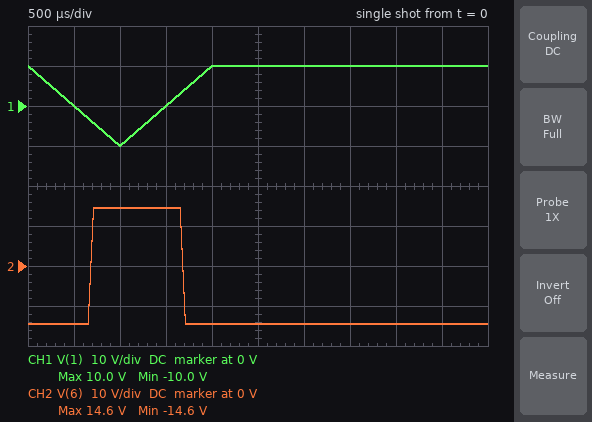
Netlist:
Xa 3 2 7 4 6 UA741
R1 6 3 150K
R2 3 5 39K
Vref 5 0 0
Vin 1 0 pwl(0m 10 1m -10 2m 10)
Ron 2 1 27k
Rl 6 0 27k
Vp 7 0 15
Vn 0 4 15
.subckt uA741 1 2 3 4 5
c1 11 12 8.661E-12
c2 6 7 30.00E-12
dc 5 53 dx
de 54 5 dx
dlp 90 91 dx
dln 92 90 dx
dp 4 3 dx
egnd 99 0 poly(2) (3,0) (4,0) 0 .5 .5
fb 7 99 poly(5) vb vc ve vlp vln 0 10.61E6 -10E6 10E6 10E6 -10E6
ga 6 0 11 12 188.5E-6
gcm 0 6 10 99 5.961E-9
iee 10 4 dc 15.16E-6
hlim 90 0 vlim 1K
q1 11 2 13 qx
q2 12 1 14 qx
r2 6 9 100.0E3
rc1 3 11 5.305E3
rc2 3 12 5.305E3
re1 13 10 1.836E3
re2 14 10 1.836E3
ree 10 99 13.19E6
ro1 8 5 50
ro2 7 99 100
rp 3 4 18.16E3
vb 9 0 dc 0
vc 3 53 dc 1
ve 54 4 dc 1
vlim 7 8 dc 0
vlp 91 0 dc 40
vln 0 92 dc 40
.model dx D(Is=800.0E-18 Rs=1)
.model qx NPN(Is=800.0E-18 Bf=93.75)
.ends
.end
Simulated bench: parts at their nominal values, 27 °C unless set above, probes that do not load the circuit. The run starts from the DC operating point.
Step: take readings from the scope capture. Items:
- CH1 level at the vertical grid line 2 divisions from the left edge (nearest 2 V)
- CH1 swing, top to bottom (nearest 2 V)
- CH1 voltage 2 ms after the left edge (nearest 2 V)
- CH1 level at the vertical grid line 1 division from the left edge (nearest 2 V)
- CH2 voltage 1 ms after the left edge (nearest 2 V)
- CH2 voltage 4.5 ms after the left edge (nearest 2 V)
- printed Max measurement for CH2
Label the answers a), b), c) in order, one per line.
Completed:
a) -10 V
b) 20 V
c) 10 V
d) 0 V
e) 14 V
f) -14 V
g) 14.6 V
